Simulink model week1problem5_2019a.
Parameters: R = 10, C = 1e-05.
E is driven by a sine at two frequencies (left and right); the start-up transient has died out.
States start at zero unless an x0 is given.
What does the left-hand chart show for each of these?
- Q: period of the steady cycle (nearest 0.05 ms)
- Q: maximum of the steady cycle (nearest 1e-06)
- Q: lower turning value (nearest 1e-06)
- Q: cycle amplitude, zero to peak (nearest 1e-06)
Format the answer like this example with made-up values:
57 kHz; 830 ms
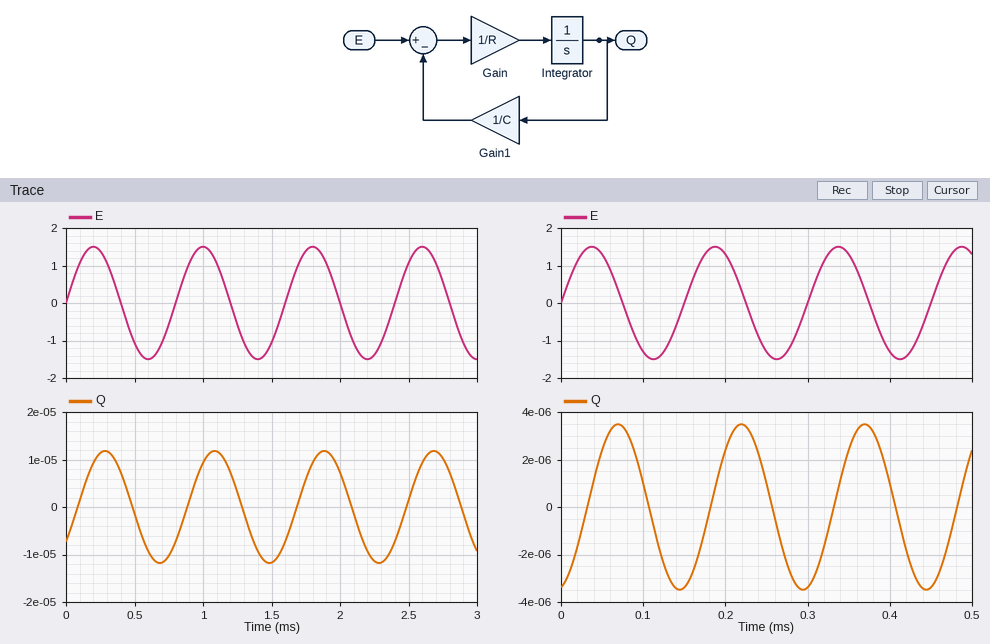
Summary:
0.80 ms; 0.000012; -0.000012; 0.000012
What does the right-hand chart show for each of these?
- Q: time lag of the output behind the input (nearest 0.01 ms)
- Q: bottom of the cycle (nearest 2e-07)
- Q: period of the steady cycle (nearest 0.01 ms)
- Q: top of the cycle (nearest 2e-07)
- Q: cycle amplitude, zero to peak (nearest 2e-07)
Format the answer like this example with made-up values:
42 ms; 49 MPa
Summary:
0.03 ms; -0.0000034; 0.15 ms; 0.0000034; 0.0000034
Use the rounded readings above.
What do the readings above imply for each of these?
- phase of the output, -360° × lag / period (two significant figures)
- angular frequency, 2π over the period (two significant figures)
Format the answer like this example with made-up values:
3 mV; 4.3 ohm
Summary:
-72°; 42 rad/ms
